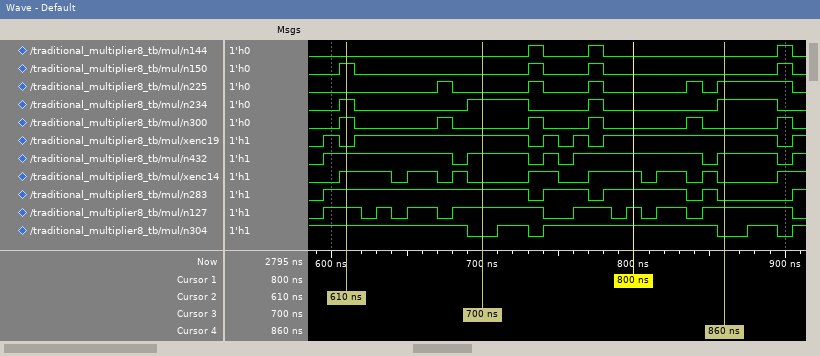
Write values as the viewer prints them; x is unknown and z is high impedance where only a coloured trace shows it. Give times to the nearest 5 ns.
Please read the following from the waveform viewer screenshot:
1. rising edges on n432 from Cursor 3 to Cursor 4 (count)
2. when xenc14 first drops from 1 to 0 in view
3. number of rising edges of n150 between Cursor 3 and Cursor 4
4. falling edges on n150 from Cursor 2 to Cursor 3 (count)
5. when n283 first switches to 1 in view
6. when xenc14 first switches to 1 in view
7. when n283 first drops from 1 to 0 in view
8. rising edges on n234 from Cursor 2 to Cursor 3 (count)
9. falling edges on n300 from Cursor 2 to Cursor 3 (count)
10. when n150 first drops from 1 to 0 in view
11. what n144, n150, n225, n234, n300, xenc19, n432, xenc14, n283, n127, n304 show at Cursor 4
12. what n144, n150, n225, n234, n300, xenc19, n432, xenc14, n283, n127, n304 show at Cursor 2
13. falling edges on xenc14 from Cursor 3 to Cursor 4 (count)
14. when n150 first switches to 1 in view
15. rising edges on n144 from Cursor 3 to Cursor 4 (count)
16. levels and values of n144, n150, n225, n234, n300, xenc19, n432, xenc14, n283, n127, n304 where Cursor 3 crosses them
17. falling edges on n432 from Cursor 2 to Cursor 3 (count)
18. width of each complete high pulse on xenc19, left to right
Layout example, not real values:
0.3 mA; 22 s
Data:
3; 640 ns; 2; 1; 595 ns; 605 ns; 730 ns; 1; 2; 615 ns; n144=0, n150=0, n225=1, n234=1, n300=0, xenc19=1, n432=1, xenc14=0, n283=0, n127=1, n304=0; n144=0, n150=1, n225=0, n234=1, n300=1, xenc19=0, n432=1, xenc14=1, n283=1, n127=1, n304=1; 4; 605 ns; 2; n144=0, n150=0, n225=0, n234=1, n300=0, xenc19=1, n432=1, xenc14=0, n283=1, n127=1, n304=0; 1; 10 ns, 115 ns, 10 ns, 10 ns, 115 ns
